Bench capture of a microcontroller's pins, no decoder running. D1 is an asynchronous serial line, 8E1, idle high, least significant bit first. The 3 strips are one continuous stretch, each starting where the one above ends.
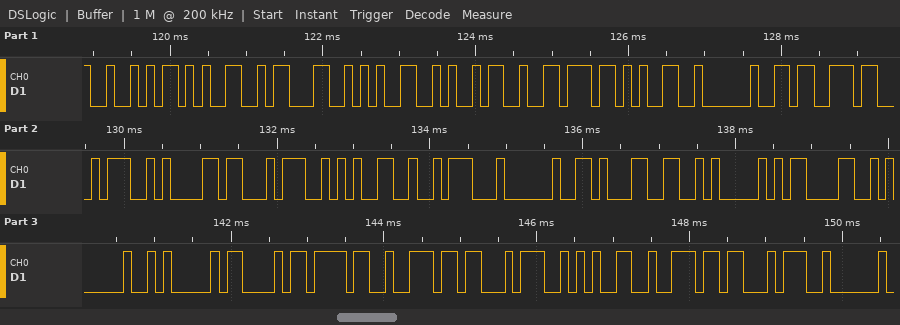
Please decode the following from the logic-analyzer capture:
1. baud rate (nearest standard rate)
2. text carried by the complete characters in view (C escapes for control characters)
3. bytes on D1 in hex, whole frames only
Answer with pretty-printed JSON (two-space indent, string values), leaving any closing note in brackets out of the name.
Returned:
{
  "baud rate": "9600 baud",
  "text carried by the complete characters in view": "\"Receive state: 1\\n\\r\\n\\nContent\"",
  "bytes on D1 in hex, whole frames only": "52 65 63 65 69 76 65 20 73 74 61 74 65 3A 20 31 0A 0D 0A 0A 43 6F 6E 74 65 6E 74"
}
